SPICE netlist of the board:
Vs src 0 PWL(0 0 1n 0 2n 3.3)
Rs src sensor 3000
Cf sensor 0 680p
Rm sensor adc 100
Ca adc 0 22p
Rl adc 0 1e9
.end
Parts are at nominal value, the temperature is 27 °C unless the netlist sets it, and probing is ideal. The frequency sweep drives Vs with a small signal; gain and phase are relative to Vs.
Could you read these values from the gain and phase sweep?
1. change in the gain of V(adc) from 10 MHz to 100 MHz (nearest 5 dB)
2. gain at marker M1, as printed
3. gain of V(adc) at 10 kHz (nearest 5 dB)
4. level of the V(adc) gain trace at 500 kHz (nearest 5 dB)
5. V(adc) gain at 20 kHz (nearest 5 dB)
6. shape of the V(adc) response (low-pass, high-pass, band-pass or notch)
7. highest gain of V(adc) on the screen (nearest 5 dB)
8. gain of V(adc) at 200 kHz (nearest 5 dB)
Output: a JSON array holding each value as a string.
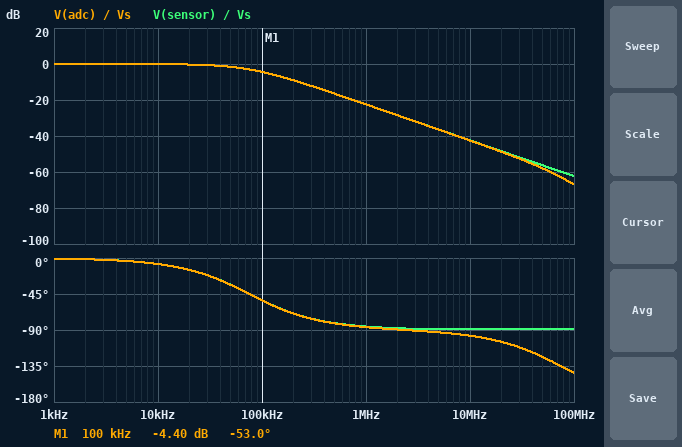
["-25 dB", "-4.40 dB", "0 dB", "-15 dB", "0 dB", "low-pass", "0 dB", "-10 dB"]
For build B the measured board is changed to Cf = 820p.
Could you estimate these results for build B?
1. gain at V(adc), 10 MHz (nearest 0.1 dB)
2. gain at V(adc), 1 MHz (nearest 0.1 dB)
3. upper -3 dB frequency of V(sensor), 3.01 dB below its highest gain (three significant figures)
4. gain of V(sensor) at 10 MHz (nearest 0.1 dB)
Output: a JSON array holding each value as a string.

["-44.1 dB", "-24.0 dB", "63.0 kHz", "-44.0 dB"]
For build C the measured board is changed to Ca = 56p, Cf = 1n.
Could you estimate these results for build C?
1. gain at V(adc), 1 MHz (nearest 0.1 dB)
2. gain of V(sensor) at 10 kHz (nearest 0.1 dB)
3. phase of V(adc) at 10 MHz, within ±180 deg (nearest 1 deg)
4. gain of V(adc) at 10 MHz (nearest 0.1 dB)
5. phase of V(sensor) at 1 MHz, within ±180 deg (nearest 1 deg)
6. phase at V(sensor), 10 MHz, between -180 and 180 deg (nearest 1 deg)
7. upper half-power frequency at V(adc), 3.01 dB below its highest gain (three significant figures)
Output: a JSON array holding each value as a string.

["-26.0 dB", "-0.2 dB", "-108 deg", "-46.4 dB", "-87 deg", "-89 deg", "50.2 kHz"]
